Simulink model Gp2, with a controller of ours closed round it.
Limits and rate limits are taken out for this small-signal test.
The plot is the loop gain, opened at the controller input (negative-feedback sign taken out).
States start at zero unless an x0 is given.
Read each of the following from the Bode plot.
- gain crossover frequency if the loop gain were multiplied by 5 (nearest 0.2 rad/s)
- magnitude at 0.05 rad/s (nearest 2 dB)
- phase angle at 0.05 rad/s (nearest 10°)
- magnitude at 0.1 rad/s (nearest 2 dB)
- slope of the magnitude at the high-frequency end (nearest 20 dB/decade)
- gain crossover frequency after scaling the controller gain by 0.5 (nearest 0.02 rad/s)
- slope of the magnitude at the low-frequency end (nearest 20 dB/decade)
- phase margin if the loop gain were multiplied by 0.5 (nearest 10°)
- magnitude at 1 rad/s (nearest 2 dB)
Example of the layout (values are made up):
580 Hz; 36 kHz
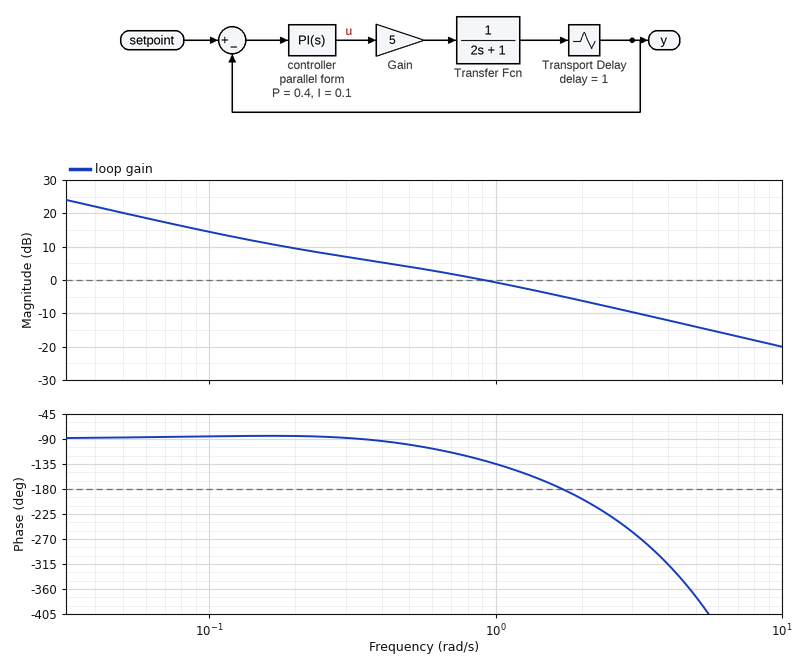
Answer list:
5.0 rad/s; 20 dB; -90°; 14 dB; -20 dB/decade; 0.36 rad/s; -20 dB/decade; 90°; 0 dB
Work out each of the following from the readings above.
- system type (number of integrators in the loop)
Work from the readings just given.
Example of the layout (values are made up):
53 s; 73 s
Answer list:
1
